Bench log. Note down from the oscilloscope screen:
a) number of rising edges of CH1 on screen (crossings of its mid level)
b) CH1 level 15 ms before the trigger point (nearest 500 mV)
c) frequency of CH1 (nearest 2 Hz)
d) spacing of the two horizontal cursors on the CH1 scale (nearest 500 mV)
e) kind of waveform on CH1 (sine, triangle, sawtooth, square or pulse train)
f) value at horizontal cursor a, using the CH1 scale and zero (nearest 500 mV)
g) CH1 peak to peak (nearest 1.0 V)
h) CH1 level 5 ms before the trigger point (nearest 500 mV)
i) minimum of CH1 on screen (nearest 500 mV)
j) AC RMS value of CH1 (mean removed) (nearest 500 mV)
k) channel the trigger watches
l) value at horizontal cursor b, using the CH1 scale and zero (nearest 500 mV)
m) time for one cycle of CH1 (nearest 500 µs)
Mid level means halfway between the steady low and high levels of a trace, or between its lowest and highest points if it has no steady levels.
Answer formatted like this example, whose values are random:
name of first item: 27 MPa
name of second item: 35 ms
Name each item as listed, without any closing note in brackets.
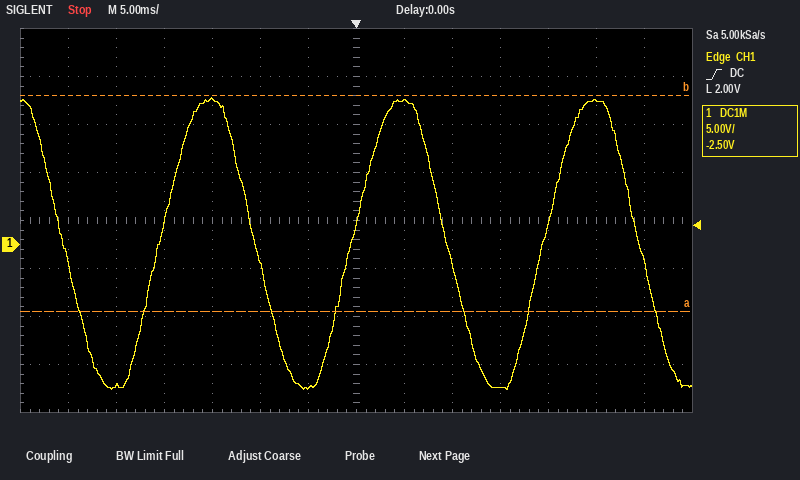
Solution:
number of rising edges of CH1 on screen: 3
CH1 level 15 ms before the trigger point: 15.0 V
frequency of CH1: 50 Hz
spacing of the two horizontal cursors on the CH1 scale: 22.5 V
kind of waveform on CH1: sine
value at horizontal cursor a, using the CH1 scale and zero: -7.0 V
CH1 peak to peak: 30.0 V
CH1 level 5 ms before the trigger point: -15.0 V
minimum of CH1 on screen: -15.0 V
AC RMS value of CH1 (mean removed): 10.5 V
channel the trigger watches: CH1
value at horizontal cursor b, using the CH1 scale and zero: 15.5 V
time for one cycle of CH1: 20.0 ms
